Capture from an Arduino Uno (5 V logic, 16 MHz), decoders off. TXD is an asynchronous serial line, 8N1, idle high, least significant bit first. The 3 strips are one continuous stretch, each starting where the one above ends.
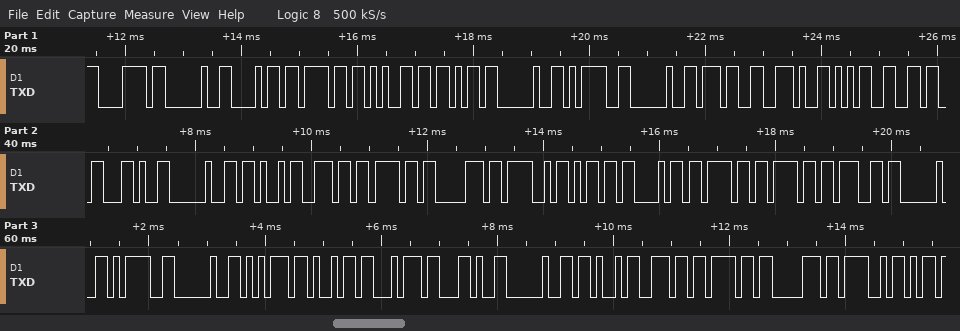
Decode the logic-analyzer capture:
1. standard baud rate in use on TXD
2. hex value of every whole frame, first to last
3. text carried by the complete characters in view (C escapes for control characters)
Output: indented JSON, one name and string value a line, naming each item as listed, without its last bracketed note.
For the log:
{
  "standard baud rate in use on TXD": "9600 baud",
  "hex value of every whole frame, first to last": "78 20 68 6F 65 6B 20 3D 20 37 2E 35 36 2C 20 4B 6E 6F 70 4F 6D 68 6F 6F 67 20 3D 20 75 69 74 2C 20 4B 6E 6F 70 4F",
  "text carried by the complete characters in view": "\"x hoek = 7.56, KnopOmhoog = uit, KnopO\""
}
